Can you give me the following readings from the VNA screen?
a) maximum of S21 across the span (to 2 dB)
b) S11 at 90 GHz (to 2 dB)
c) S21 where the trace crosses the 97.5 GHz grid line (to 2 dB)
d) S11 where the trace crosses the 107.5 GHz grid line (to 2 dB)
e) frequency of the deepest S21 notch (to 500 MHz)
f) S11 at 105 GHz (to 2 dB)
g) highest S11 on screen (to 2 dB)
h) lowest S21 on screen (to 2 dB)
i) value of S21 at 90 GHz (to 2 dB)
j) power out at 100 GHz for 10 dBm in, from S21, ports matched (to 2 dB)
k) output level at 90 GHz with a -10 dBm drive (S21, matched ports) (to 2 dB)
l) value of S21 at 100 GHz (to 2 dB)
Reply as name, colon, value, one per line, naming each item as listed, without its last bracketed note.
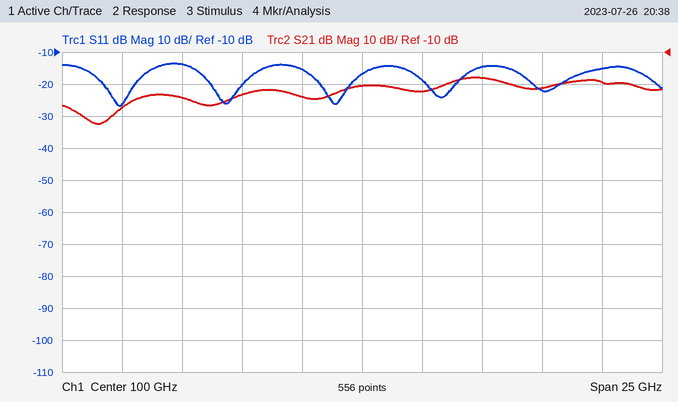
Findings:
maximum of S21 across the span: -18 dB
S11 at 90 GHz: -26 dB
S21 where the trace crosses the 97.5 GHz grid line: -24 dB
S11 where the trace crosses the 107.5 GHz grid line: -22 dB
frequency of the deepest S21 notch: 89.0 GHz
S11 at 105 GHz: -14 dB
highest S11 on screen: -14 dB
lowest S21 on screen: -32 dB
value of S21 at 90 GHz: -28 dB
power out at 100 GHz for 10 dBm in, from S21, ports matched: -10 dBm
output level at 90 GHz with a -10 dBm drive (S21, matched ports): -38 dBm
value of S21 at 100 GHz: -20 dB
